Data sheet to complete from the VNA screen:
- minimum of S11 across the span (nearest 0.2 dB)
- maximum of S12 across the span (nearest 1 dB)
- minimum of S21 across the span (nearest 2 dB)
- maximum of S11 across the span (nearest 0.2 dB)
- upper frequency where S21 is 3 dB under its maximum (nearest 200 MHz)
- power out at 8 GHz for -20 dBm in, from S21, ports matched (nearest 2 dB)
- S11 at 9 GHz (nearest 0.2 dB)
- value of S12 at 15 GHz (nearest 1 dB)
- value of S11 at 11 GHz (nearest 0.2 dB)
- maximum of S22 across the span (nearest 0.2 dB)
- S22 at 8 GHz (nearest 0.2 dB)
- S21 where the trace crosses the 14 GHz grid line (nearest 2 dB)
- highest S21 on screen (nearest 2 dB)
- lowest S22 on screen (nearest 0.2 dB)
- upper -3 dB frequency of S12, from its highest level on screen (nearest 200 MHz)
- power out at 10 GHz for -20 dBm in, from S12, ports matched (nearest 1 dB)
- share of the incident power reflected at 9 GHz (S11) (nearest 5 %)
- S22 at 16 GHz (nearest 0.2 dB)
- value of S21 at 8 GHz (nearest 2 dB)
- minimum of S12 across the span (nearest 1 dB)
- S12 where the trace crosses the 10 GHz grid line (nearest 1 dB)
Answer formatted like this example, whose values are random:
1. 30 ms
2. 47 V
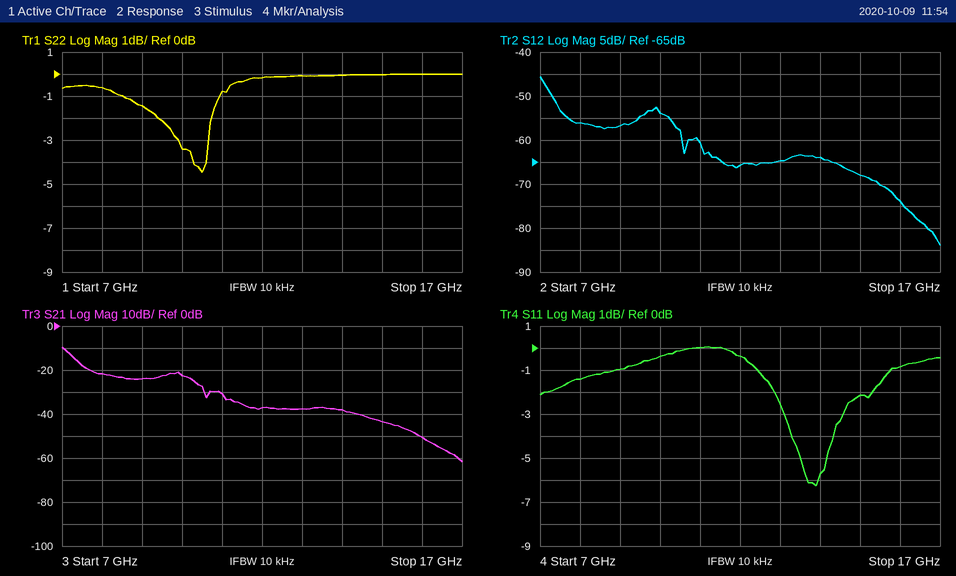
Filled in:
1. -6.2 dB
2. -46 dB
3. -62 dB
4. 0.0 dB
5. 7.2 GHz
6. -42 dBm
7. -1.0 dB
8. -68 dB
9. 0.0 dB
10. 0.0 dB
11. -0.6 dB
12. -38 dB
13. -10 dB
14. -4.4 dB
15. 7.2 GHz
16. -74 dBm
17. 80 %
18. 0.0 dB
19. -22 dB
20. -84 dB
21. -54 dB
